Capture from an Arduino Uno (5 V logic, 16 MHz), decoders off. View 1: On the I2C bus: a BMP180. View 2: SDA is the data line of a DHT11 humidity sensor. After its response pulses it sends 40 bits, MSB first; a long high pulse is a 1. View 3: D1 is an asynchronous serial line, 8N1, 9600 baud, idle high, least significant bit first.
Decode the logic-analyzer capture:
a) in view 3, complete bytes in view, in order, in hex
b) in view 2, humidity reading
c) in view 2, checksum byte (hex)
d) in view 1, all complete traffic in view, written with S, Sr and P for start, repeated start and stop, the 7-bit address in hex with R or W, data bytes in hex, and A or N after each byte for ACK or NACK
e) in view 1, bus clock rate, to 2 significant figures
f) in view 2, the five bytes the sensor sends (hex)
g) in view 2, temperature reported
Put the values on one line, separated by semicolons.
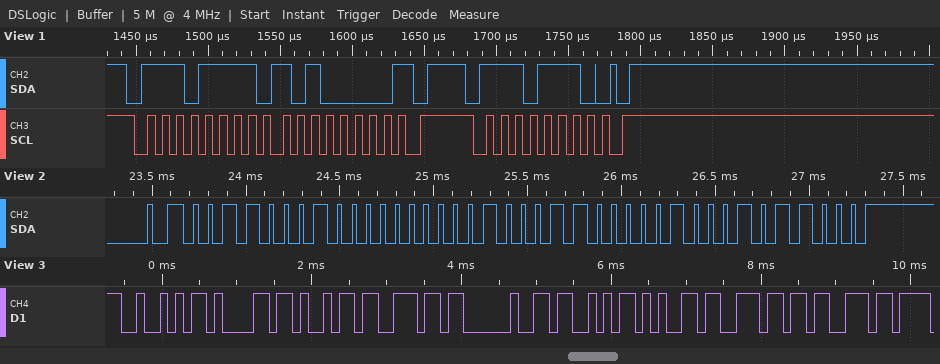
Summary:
52 61 69 6E 20 53 65 6E 73; 49 %; 0x58; S 77R A A0 N P S 77W A P; 100 kHz; 31 00 23 04 58; 35.4 °C
